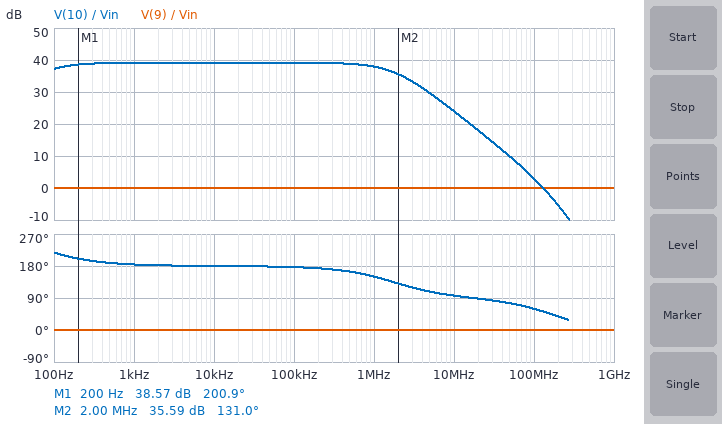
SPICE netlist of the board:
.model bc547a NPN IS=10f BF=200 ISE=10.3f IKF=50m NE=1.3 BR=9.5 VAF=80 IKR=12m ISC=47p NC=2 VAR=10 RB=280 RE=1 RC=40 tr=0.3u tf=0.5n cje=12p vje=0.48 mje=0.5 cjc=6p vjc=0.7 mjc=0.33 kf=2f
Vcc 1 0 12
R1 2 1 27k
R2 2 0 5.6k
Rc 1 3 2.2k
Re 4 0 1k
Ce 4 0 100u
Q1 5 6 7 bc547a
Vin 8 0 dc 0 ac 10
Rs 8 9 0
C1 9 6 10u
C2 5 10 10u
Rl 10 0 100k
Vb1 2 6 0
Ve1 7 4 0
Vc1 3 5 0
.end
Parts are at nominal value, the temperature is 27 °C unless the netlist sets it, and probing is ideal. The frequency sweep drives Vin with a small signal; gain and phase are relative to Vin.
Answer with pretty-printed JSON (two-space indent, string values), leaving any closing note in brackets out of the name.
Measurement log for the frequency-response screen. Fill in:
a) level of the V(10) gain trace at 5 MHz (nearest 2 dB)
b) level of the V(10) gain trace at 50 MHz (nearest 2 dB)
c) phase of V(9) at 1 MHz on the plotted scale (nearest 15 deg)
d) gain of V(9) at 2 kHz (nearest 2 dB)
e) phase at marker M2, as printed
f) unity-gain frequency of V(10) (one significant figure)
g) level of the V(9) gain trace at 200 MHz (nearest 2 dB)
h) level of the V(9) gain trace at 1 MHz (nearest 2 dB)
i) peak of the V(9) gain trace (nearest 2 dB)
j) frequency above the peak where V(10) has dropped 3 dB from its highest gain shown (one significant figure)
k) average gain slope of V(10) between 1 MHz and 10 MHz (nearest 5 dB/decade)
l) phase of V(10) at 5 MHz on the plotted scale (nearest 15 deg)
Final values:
{
  "level of the V(10) gain trace at 5 MHz": "30 dB",
  "level of the V(10) gain trace at 50 MHz": "10 dB",
  "phase of V(9) at 1 MHz on the plotted scale": "0 deg",
  "gain of V(9) at 2 kHz": "0 dB",
  "phase at marker M2, as printed": "131.0 deg",
  "unity-gain frequency of V(10)": "100 MHz",
  "level of the V(9) gain trace at 200 MHz": "0 dB",
  "level of the V(9) gain trace at 1 MHz": "0 dB",
  "peak of the V(9) gain trace": "0 dB",
  "frequency above the peak where V(10) has dropped 3 dB from its highest gain shown": "2 MHz",
  "average gain slope of V(10) between 1 MHz and 10 MHz": "-15 dB/decade",
  "phase of V(10) at 5 MHz on the plotted scale": "105 deg"
}
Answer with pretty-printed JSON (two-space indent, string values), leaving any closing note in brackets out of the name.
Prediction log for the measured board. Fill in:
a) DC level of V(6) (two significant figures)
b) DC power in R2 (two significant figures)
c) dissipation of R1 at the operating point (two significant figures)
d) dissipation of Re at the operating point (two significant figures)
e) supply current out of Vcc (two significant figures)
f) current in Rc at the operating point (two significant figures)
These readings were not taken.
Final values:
{
  "DC level of V(6)": "2.0 V",
  "DC power in R2": "720 µW",
  "dissipation of R1 at the operating point": "3.7 mW",
  "dissipation of Re at the operating point": "1.8 mW",
  "supply current out of Vcc": "1.7 mA",
  "current in Rc at the operating point": "1.3 mA"
}
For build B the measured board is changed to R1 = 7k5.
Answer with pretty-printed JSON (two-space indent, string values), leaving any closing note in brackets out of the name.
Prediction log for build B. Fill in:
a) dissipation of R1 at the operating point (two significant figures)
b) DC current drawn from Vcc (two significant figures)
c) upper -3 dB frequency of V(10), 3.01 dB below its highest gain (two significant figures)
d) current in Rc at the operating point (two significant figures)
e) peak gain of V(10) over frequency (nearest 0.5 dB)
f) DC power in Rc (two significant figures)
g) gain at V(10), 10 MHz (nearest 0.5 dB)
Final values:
{
  "dissipation of R1 at the operating point": "7.4 mW",
  "DC current drawn from Vcc": "4.6 mA",
  "upper -3 dB frequency of V(10), 3.01 dB below its highest gain": "75 kHz",
  "current in Rc at the operating point": "3.6 mA",
  "peak gain of V(10) over frequency": "-8.0 dB",
  "DC power in Rc": "29 mW",
  "gain at V(10), 10 MHz": "-32.5 dB"
}
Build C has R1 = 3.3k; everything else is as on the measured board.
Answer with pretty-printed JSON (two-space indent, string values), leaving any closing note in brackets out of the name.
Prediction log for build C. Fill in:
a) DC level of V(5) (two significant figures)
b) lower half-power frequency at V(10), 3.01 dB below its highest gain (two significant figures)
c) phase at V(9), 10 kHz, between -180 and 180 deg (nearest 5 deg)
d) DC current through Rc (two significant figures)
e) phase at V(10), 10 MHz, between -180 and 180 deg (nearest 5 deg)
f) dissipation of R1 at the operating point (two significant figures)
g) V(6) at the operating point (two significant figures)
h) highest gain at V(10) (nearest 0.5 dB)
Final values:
{
  "DC level of V(5)": "4.6 V",
  "lower half-power frequency at V(10), 3.01 dB below its highest gain": "2.6 Hz",
  "phase at V(9), 10 kHz, between -180 and 180 deg": "0 deg",
  "DC current through Rc": "3.4 mA",
  "phase at V(10), 10 MHz, between -180 and 180 deg": "0 deg",
  "dissipation of R1 at the operating point": "13 mW",
  "V(6) at the operating point": "5.4 V",
  "highest gain at V(10)": "-22.5 dB"
}
